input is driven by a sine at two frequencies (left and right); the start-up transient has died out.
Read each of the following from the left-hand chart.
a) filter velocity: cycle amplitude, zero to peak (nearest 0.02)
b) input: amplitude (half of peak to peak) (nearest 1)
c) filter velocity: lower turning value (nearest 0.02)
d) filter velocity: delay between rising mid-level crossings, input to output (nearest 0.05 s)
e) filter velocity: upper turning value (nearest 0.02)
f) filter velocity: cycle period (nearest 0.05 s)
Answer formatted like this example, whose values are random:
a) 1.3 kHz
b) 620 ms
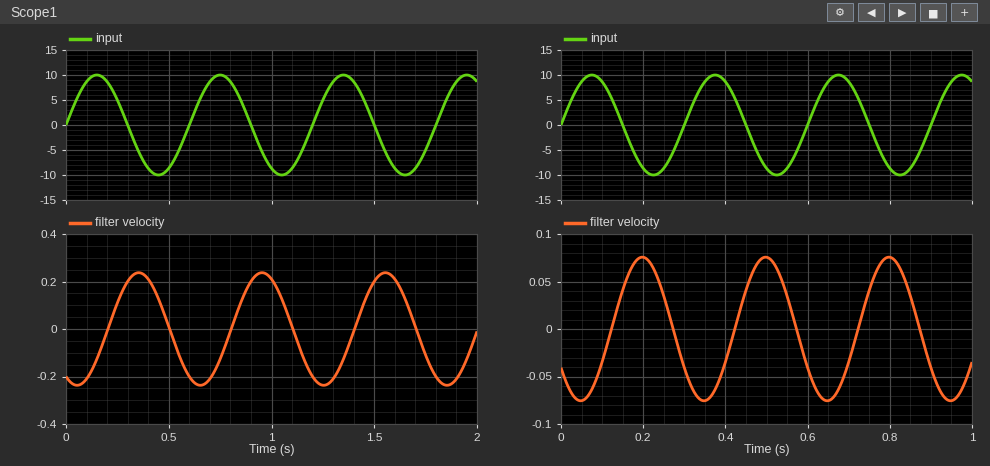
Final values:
a) 0.24
b) 10
c) -0.24
d) 0.20 s
e) 0.24
f) 0.60 s
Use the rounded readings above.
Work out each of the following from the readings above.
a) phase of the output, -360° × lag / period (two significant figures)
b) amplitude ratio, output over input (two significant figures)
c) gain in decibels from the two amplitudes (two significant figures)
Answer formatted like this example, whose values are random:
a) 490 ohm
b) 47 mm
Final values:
a) -120°
b) 0.024
c) -32 dB
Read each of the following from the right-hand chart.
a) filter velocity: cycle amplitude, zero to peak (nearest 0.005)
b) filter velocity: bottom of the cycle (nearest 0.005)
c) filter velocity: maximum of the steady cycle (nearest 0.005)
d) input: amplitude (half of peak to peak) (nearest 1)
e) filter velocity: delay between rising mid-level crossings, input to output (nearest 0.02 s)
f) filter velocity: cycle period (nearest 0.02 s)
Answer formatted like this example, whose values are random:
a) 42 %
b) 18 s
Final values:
a) 0.075
b) -0.075
c) 0.075
d) 10
e) 0.12 s
f) 0.30 s
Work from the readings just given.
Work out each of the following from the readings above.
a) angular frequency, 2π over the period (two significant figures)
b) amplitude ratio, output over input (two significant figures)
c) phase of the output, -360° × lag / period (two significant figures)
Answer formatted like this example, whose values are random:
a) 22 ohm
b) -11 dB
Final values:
a) 21 rad/s
b) 0.0075
c) -140°
